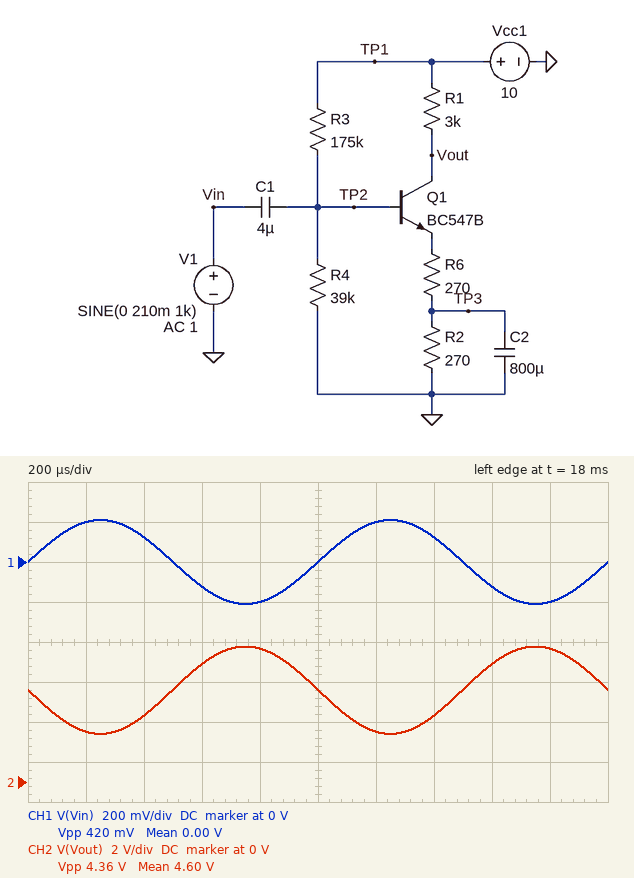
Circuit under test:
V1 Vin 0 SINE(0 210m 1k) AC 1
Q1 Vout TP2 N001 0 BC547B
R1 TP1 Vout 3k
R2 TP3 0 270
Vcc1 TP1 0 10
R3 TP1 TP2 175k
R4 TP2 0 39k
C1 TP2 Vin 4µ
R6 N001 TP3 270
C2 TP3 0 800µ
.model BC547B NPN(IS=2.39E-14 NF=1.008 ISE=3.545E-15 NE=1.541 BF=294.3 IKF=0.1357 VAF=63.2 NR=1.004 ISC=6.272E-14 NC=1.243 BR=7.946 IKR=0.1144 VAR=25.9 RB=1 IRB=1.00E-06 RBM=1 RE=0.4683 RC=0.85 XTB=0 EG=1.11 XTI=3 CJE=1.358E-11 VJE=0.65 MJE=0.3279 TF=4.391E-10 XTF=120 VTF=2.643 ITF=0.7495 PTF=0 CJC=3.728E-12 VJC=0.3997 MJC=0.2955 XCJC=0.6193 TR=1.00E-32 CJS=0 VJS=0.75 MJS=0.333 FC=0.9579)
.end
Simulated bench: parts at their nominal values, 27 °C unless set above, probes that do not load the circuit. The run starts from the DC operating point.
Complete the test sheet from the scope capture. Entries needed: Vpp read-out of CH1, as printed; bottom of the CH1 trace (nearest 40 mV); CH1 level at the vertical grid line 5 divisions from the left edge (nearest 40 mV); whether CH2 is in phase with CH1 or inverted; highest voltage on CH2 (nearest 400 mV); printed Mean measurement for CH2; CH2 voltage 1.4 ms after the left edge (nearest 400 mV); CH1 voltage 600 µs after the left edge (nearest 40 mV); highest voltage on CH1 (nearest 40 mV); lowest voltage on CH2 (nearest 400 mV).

420 mV
-200 mV
0 V
inverted
6.8 V
4.60 V
3.2 V
-120 mV
200 mV
2.4 V
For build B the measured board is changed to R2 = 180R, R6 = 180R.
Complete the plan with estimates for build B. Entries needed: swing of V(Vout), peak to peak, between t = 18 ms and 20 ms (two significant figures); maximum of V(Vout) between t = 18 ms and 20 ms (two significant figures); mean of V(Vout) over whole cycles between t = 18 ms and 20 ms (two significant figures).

6.1 V
7.1 V
4.0 V
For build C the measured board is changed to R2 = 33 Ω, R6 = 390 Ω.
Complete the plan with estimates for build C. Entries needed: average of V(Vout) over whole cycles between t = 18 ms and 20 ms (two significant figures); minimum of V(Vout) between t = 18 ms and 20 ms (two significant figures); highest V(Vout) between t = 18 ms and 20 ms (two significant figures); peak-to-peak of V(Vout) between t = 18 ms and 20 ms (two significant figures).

3.5 V
1.9 V
5.0 V
3.1 V
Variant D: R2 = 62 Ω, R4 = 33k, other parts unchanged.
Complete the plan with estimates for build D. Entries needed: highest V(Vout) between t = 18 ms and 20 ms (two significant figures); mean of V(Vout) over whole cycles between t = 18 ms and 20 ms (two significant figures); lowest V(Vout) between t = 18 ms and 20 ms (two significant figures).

5.7 V
3.5 V
1.3 V
